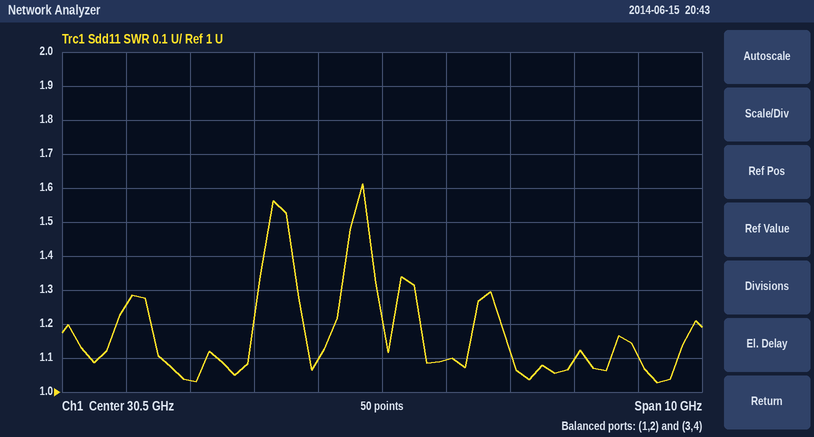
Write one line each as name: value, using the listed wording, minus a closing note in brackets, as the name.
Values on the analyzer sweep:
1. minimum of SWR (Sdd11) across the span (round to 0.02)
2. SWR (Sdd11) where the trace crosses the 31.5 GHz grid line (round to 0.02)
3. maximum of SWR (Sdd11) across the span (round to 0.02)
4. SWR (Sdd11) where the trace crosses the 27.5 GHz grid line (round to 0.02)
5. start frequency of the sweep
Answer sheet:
minimum of SWR (Sdd11) across the span: 1.02
SWR (Sdd11) where the trace crosses the 31.5 GHz grid line: 1.10
maximum of SWR (Sdd11) across the span: 1.62
SWR (Sdd11) where the trace crosses the 27.5 GHz grid line: 1.04
start frequency of the sweep: 25.5 GHz
